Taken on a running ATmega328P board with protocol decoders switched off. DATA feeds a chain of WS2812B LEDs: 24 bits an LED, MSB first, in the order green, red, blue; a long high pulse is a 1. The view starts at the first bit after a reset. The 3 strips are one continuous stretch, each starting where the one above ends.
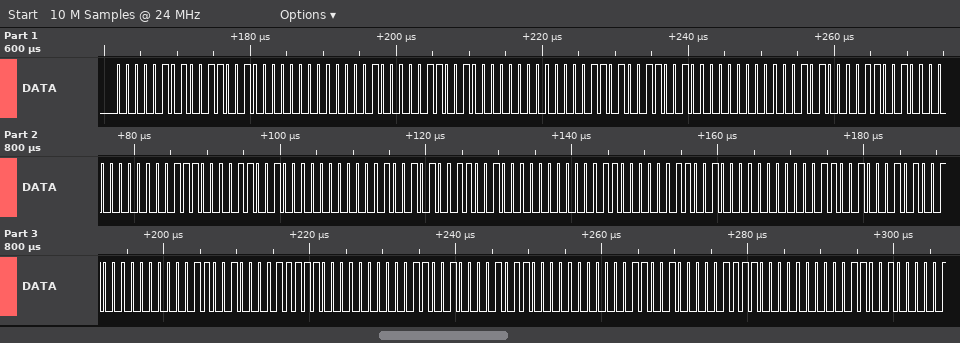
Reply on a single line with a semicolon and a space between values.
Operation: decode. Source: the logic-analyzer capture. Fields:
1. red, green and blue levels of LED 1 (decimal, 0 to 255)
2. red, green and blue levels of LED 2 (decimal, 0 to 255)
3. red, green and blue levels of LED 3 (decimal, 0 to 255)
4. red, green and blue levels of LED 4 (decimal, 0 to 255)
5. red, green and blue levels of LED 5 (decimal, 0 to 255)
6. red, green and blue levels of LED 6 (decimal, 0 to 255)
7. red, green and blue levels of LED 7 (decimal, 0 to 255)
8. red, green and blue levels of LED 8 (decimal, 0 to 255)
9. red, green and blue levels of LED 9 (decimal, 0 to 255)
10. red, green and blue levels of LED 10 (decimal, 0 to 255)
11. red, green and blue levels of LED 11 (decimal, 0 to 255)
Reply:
50, 5, 0; 50, 8, 0; 50, 13, 0; 50, 20, 0; 50, 28, 0; 50, 37, 0; 50, 48, 0; 41, 50, 0; 31, 50, 0; 22, 50, 0; 15, 50, 0
